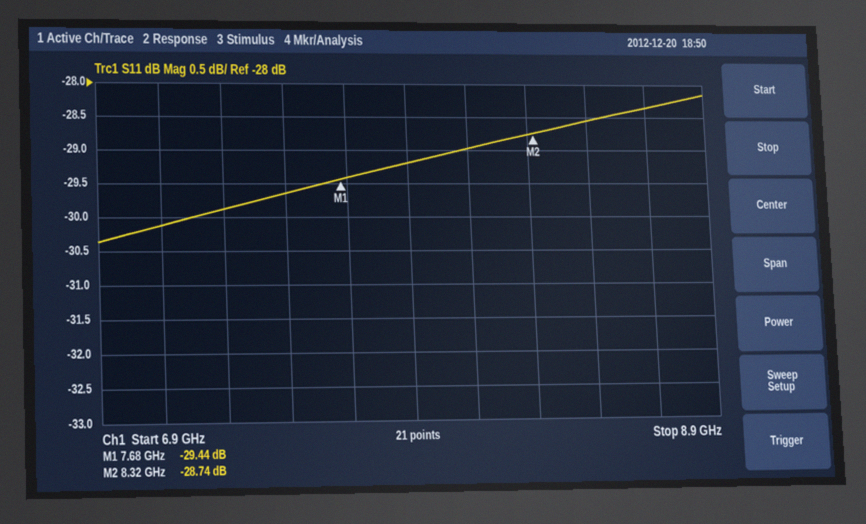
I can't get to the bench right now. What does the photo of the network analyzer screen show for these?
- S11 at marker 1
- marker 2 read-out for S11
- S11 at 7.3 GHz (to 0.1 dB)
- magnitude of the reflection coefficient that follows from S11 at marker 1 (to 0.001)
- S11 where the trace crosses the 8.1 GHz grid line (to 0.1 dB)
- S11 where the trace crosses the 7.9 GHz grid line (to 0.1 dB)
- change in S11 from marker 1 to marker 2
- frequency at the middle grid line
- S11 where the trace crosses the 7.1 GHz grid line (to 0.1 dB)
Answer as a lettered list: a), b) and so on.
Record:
a) -29.44 dB
b) -28.74 dB
c) -29.9 dB
d) 0.034
e) -29.0 dB
f) -29.2 dB
g) 0.70 dB
h) 7.9 GHz
i) -30.1 dB
